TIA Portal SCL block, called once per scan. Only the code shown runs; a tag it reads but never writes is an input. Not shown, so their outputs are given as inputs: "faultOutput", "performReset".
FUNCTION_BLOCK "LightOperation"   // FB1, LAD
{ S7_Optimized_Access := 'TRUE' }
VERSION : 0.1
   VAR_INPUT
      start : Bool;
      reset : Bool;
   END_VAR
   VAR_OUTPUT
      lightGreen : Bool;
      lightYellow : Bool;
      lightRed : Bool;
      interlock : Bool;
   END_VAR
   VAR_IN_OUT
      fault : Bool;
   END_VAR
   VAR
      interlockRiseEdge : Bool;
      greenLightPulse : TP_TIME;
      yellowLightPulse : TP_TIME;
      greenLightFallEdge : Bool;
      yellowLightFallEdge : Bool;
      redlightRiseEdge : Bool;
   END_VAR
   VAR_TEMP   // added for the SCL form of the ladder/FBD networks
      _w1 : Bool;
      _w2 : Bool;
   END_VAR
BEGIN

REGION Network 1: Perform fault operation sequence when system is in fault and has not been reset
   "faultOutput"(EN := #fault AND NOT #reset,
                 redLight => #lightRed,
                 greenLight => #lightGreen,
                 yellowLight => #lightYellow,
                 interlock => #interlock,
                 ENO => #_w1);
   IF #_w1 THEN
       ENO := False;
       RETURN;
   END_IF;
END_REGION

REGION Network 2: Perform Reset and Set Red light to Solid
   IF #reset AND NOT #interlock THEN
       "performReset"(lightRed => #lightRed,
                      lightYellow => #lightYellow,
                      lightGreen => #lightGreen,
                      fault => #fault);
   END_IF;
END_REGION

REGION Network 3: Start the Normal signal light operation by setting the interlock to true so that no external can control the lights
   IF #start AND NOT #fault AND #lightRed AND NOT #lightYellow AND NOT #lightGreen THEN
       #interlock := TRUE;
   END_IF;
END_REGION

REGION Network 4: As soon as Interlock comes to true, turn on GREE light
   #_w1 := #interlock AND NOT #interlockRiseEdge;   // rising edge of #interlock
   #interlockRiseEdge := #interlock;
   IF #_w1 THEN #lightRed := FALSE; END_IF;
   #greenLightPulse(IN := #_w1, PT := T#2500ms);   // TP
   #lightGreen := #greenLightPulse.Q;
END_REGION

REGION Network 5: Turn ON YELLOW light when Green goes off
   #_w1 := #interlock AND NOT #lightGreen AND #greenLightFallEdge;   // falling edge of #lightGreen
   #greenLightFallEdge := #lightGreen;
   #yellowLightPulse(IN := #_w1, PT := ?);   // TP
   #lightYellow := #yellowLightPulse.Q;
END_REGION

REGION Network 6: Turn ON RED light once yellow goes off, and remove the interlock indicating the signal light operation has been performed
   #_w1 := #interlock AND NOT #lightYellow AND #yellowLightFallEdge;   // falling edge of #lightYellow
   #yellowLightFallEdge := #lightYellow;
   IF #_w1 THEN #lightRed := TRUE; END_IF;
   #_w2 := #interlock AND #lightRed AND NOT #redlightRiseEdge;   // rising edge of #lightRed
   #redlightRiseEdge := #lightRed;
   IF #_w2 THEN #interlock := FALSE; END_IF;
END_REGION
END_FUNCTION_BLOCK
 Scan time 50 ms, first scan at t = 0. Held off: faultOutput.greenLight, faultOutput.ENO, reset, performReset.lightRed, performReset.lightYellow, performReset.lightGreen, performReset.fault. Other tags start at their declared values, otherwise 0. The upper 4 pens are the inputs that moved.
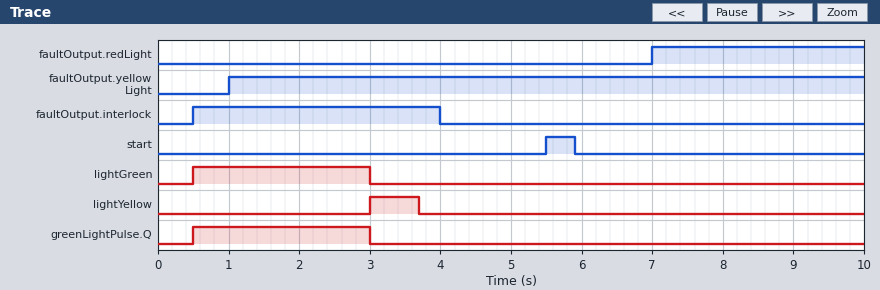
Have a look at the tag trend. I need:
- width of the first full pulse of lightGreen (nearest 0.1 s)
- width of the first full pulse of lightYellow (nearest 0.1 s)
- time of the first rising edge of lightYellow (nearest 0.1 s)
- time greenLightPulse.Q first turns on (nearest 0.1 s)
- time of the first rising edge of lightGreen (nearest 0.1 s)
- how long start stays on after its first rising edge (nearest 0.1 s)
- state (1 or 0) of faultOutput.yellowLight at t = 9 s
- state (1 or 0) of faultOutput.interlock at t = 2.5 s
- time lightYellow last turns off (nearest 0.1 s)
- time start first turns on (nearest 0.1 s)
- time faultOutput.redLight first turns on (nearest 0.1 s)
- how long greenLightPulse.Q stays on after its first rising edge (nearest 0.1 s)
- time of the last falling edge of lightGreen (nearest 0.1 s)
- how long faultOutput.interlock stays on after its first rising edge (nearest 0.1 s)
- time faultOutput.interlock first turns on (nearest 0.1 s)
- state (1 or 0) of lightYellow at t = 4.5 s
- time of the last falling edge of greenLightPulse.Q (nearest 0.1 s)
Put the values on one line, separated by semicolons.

2.5 s; 0.7 s; 3.0 s; 0.5 s; 0.5 s; 0.4 s; 1; 1; 3.7 s; 5.5 s; 7.0 s; 2.5 s; 3.0 s; 3.5 s; 0.5 s; 0; 3.0 s
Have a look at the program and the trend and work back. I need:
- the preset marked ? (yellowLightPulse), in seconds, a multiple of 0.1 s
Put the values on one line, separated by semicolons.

0.7 s
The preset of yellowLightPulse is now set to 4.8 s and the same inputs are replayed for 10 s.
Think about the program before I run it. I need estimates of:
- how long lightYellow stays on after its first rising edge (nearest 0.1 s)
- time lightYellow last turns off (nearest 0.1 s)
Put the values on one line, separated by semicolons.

4.8 s; 7.8 s
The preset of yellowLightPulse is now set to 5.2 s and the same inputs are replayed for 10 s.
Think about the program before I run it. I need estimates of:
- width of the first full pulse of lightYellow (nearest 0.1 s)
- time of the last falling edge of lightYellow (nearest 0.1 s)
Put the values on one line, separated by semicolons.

5.2 s; 8.2 s
